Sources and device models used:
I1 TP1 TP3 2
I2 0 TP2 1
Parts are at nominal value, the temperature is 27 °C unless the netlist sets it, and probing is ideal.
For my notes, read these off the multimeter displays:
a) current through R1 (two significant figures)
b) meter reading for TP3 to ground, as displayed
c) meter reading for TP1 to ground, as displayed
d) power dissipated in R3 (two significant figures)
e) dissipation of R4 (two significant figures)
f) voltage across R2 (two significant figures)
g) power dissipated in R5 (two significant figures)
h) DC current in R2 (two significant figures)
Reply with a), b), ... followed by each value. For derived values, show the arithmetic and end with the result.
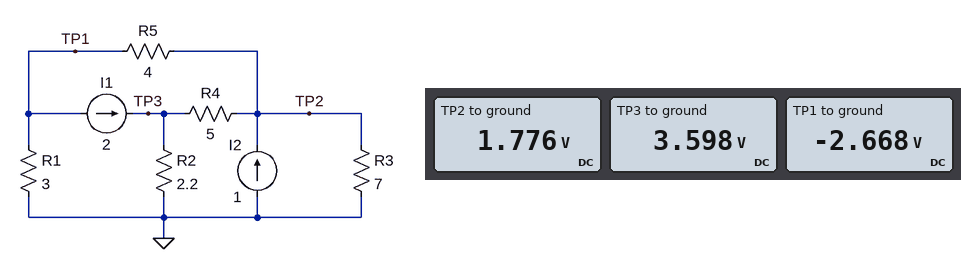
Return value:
a) (0 V - (-2.668 V)) / 3 Ω = 890 mA
b) 3.598 V
c) -2.668 V
d) (1.776 V)^2 / 7 Ω = 450 mW
e) (3.598 V - 1.776 V)^2 / 5 Ω = 660 mW
f) 3.598 V = 3.6 V
g) (1.776 V - (-2.668 V))^2 / 4 Ω = 4.9 W
h) (3.598 V) / 2.2 Ω = 1.6 A
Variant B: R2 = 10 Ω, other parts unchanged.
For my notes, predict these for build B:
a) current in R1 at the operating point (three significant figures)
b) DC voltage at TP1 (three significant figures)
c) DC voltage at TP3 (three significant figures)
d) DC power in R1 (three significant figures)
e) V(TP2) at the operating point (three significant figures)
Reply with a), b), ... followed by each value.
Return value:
a) 544 mA
b) -1.63 V
c) 9.46 V
d) 889 mW
e) 4.19 V
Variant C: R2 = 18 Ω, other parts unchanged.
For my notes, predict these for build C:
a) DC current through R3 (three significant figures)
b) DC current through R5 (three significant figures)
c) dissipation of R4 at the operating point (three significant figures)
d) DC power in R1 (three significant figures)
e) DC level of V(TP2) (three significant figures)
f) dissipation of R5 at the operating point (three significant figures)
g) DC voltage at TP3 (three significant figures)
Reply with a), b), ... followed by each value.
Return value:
a) 741 mA
b) 1.60 A
c) 8.97 W
d) 484 mW
e) 5.19 V
f) 10.2 W
g) 11.9 V
